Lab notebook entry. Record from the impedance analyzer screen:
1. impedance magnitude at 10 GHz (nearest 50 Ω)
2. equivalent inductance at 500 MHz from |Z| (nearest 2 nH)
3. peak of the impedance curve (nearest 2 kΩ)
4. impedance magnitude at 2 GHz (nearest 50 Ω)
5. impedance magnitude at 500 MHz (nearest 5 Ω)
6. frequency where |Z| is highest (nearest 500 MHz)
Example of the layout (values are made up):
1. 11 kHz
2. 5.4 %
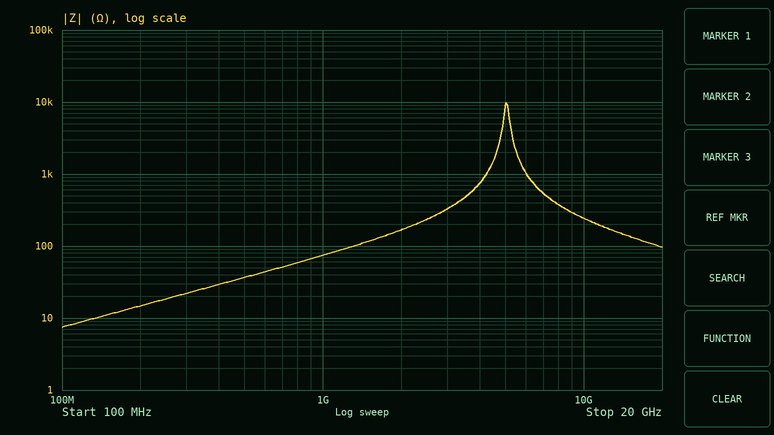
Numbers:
1. 250 Ω
2. 12 nH
3. 10 kΩ
4. 150 Ω
5. 35 Ω
6. 5.0 GHz
